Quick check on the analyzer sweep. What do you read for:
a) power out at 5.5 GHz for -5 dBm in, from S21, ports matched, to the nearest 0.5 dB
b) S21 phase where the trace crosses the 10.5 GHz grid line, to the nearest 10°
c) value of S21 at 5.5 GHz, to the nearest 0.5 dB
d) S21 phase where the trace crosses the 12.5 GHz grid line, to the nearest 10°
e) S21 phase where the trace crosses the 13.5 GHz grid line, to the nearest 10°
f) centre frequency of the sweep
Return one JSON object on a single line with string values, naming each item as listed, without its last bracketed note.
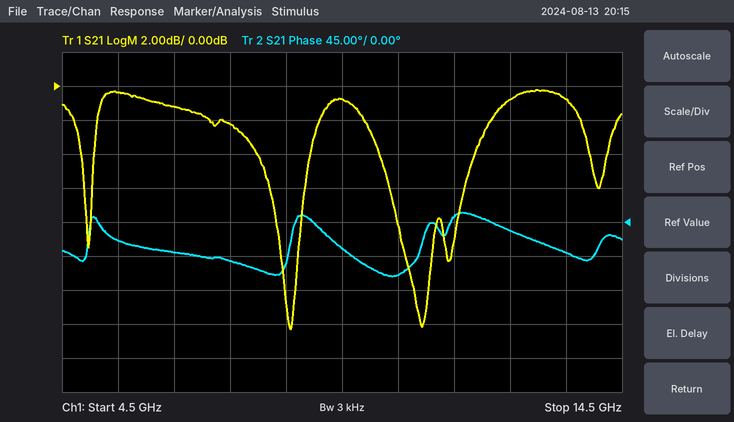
{"power out at 5.5 GHz for -5 dBm in, from S21, ports matched, to the nearest 0.5 dB": "-5.5 dBm", "S21 phase where the trace crosses the 10.5 GHz grid line, to the nearest 10°": "-70°", "value of S21 at 5.5 GHz, to the nearest 0.5 dB": "-0.5 dB", "S21 phase where the trace crosses the 12.5 GHz grid line, to the nearest 10°": "-10°", "S21 phase where the trace crosses the 13.5 GHz grid line, to the nearest 10°": "-40°", "centre frequency of the sweep": "9.5 GHz"}
